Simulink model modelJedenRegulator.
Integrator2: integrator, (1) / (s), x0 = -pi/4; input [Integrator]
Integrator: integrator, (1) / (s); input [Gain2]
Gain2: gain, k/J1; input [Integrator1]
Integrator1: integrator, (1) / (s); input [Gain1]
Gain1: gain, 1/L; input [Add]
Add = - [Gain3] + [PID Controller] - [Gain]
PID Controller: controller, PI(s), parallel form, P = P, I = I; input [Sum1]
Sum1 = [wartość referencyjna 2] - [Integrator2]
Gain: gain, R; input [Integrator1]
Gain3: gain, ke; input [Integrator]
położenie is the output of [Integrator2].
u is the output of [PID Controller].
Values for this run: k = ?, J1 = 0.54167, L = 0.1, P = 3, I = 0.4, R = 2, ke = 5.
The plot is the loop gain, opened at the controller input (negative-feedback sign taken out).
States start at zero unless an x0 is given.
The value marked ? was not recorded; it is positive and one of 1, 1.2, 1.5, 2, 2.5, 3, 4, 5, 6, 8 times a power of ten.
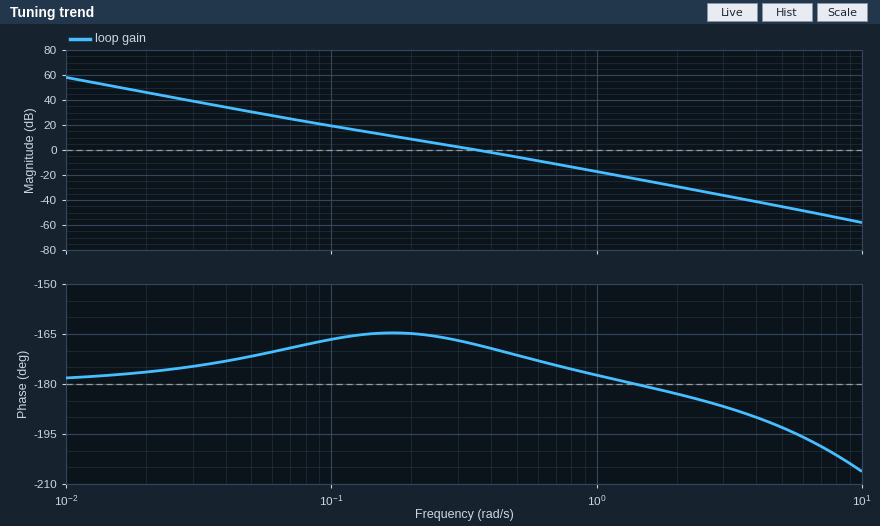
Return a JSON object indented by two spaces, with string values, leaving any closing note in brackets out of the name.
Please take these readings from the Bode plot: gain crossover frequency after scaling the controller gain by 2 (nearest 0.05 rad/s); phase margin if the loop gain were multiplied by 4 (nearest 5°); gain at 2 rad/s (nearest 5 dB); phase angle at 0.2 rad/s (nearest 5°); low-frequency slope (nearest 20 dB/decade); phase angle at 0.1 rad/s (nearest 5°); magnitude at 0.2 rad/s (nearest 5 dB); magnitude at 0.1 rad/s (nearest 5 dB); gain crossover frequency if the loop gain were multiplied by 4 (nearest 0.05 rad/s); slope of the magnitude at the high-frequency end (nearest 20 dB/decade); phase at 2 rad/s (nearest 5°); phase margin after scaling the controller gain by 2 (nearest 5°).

{
  "gain crossover frequency after scaling the controller gain by 2": "0.50 rad/s",
  "phase margin if the loop gain were multiplied by 4": "5°",
  "gain at 2 rad/s": "-30 dB",
  "phase angle at 0.2 rad/s": "-165°",
  "low-frequency slope": "-40 dB/decade",
  "phase angle at 0.1 rad/s": "-165°",
  "magnitude at 0.2 rad/s": "10 dB",
  "magnitude at 0.1 rad/s": "20 dB",
  "gain crossover frequency if the loop gain were multiplied by 4": "0.75 rad/s",
  "slope of the magnitude at the high-frequency end": "-40 dB/decade",
  "phase at 2 rad/s": "-185°",
  "phase margin after scaling the controller gain by 2": "10°"
}
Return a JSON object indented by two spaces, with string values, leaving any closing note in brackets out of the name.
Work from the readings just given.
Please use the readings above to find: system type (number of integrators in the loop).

{
  "system type": "2"
}
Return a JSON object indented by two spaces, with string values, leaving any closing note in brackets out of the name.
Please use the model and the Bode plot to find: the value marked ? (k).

{
  "the value marked ?": "0.05"
}
